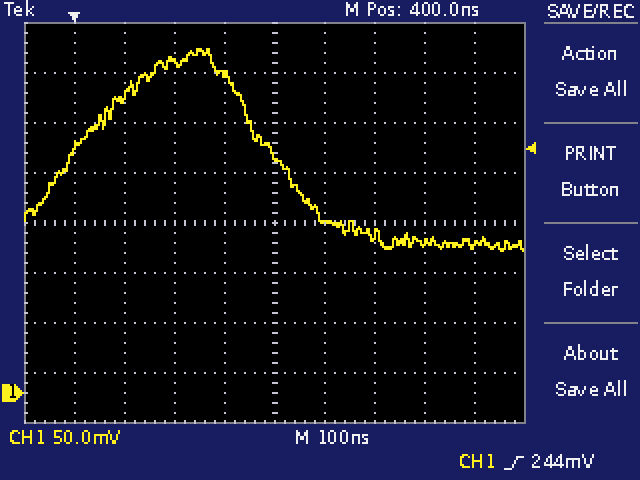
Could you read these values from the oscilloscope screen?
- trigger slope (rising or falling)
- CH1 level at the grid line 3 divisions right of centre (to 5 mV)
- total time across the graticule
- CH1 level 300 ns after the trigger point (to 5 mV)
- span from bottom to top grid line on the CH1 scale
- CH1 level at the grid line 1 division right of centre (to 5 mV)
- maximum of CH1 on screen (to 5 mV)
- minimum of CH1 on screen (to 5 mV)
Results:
rising
150 mV
1 µs
320 mV
400 mV
170 mV
345 mV
140 mV
